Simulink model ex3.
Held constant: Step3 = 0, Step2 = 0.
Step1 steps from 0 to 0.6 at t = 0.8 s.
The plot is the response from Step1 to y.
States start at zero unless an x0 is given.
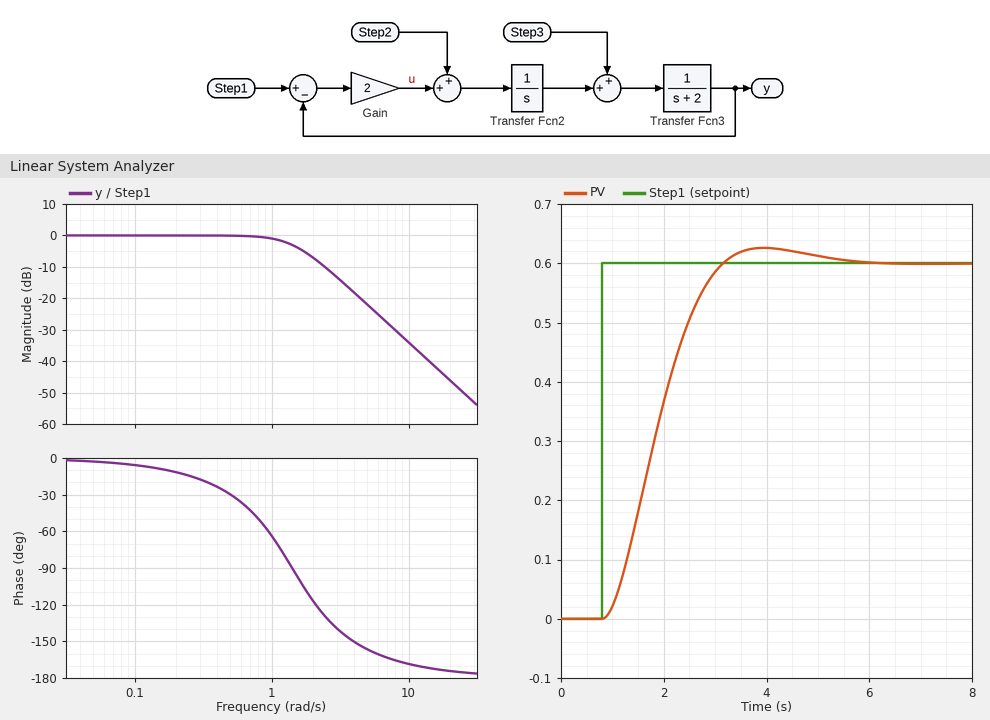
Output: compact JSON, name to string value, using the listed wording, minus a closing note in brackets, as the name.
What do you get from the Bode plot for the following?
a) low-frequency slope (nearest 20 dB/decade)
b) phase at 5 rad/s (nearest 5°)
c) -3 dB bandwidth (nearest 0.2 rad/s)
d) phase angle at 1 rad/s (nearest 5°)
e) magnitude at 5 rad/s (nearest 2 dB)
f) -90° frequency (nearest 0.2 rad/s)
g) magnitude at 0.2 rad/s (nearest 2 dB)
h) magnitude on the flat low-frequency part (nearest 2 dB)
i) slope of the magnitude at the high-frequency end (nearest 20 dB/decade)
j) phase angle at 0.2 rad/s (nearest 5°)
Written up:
{"low-frequency slope": "0 dB/decade", "phase at 5 rad/s": "-155°", "-3 dB bandwidth": "1.4 rad/s", "phase angle at 1 rad/s": "-65°", "magnitude at 5 rad/s": "-22 dB", "-90° frequency": "1.4 rad/s", "magnitude at 0.2 rad/s": "0 dB", "magnitude on the flat low-frequency part": "0 dB", "slope of the magnitude at the high-frequency end": "-40 dB/decade", "phase angle at 0.2 rad/s": "-10°"}
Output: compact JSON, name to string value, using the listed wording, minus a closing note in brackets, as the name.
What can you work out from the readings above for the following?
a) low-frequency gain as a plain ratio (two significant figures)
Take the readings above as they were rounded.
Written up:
{"low-frequency gain as a plain ratio": "1.0"}
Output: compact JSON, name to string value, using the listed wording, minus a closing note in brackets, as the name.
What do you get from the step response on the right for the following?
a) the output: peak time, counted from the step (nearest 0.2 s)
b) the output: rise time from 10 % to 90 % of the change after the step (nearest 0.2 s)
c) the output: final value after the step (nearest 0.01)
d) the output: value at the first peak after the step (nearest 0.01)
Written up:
{"the output: peak time, counted from the step": "3.2 s", "the output: rise time from 10 % to 90 % of the change after the step": "1.6 s", "the output: final value after the step": "0.60", "the output: value at the first peak after the step": "0.63"}
